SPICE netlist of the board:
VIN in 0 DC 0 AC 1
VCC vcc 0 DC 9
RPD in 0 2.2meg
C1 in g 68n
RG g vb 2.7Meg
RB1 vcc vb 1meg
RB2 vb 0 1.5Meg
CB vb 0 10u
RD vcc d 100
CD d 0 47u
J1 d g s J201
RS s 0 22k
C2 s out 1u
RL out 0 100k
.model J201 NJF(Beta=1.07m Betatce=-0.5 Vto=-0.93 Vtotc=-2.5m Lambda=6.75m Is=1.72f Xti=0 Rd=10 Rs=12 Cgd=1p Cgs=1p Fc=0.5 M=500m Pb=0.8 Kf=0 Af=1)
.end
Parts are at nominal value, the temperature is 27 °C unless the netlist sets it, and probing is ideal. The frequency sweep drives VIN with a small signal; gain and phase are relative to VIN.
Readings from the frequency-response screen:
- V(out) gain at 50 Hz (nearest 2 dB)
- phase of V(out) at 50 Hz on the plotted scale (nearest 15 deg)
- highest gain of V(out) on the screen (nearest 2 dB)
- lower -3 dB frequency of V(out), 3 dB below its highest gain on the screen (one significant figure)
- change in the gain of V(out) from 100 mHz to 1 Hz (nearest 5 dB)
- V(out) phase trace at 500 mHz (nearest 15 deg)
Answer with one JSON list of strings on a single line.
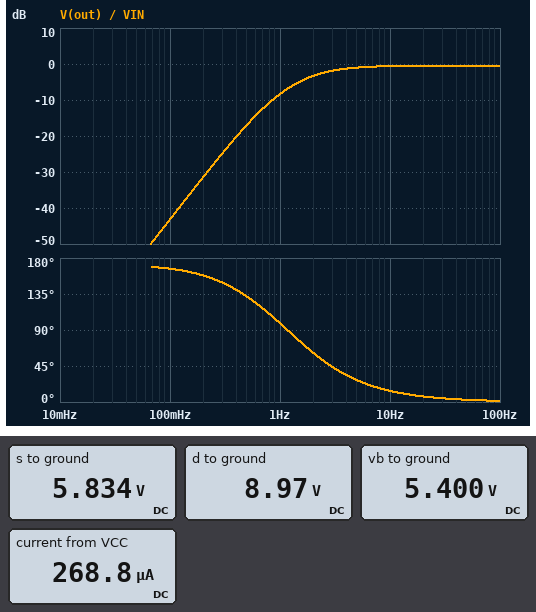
["0 dB", "0 deg", "0 dB", "2 Hz", "35 dB", "135 deg"]
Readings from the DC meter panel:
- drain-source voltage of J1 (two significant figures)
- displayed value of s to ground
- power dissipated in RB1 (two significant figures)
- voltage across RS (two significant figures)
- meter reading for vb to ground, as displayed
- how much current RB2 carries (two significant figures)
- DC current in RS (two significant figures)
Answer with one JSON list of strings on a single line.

["3.1 V", "5.834 V", "13 µW", "5.8 V", "5.400 V", "3.6 µA", "270 µA"]
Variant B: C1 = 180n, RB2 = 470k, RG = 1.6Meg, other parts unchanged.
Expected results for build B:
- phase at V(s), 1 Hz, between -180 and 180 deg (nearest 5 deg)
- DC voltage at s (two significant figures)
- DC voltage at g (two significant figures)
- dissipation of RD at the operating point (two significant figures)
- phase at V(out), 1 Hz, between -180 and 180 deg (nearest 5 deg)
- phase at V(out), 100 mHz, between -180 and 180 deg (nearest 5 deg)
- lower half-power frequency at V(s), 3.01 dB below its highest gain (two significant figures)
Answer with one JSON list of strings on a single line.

["30 deg", "3.4 V", "2.9 V", "2.4 µW", "85 deg", "160 deg", "550 mHz"]
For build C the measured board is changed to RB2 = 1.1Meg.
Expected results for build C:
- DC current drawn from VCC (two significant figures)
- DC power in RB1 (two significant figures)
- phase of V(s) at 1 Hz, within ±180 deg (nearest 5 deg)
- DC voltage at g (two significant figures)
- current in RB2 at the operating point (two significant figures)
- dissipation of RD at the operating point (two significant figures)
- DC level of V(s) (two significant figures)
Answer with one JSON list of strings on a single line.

["240 µA", "18 µW", "40 deg", "4.7 V", "4.3 µA", "5.5 µW", "5.2 V"]
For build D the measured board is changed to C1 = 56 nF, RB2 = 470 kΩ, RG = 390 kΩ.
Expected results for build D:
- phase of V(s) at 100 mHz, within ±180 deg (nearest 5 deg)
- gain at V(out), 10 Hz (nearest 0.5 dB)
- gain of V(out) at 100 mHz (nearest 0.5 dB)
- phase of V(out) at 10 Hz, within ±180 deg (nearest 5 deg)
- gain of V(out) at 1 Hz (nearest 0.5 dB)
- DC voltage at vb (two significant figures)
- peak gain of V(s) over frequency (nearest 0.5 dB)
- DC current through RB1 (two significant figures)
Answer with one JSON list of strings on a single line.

["75 deg", "-2.5 dB", "-60.0 dB", "45 deg", "-23.5 dB", "2.9 V", "-0.5 dB", "6.1 µA"]
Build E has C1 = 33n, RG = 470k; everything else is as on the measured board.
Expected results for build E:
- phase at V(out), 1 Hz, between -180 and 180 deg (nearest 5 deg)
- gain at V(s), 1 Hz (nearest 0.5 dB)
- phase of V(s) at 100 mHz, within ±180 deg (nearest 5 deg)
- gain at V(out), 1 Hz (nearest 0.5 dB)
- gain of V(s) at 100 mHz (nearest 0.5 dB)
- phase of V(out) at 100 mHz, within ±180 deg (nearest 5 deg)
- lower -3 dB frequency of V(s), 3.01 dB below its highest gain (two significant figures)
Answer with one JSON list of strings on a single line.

["140 deg", "-20.5 dB", "75 deg", "-26.0 dB", "-39.5 dB", "160 deg", "10 Hz"]
